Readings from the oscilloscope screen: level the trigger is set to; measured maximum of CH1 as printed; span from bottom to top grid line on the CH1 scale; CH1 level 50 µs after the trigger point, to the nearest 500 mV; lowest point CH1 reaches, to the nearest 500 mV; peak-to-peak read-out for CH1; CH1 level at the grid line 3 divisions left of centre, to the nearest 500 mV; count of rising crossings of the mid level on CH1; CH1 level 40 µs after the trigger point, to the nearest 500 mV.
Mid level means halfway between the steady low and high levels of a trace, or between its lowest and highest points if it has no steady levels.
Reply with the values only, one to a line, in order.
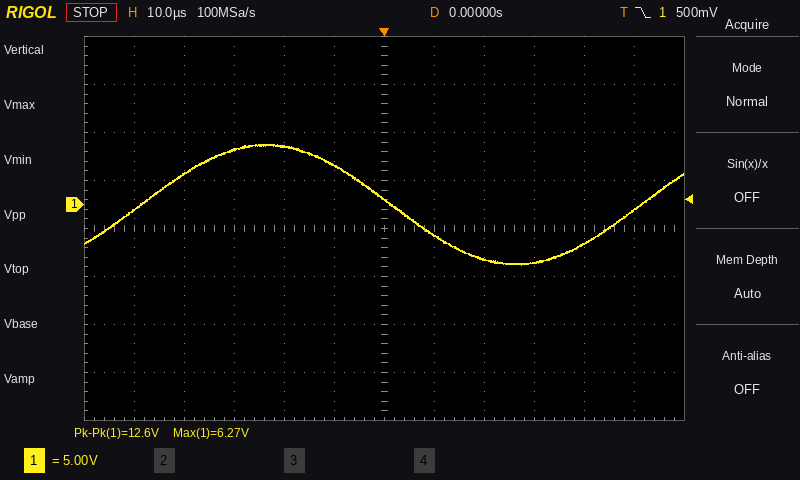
500 mV
6.27 V
40 V
-500 mV
-6.5 V
12.6 V
5.5 V
2
-4.0 V
